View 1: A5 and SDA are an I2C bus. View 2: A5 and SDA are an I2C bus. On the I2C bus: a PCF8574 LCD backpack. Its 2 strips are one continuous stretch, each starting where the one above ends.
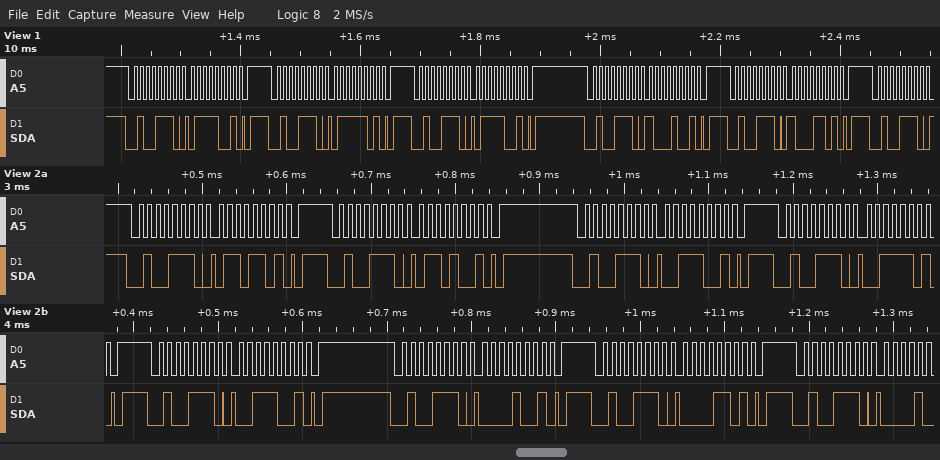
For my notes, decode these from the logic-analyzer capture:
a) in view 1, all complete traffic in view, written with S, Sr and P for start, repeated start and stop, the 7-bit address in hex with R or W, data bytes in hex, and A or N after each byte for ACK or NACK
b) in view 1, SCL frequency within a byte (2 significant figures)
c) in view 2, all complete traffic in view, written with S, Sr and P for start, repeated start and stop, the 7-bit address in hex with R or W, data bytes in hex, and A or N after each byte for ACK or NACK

S 27W A 79 A P S 27W A 7D A P S 27W A 79 A P S 27W A 89 A P S 27W A 8D A P S 27W A
100 kHz
S 27W A 6D A P S 27W A 69 A P S 27W A 39 A P S 27W A 3D A P S 27W A 39 A P S 27W A 09 A P S 27W A 0D A P S 27W A
